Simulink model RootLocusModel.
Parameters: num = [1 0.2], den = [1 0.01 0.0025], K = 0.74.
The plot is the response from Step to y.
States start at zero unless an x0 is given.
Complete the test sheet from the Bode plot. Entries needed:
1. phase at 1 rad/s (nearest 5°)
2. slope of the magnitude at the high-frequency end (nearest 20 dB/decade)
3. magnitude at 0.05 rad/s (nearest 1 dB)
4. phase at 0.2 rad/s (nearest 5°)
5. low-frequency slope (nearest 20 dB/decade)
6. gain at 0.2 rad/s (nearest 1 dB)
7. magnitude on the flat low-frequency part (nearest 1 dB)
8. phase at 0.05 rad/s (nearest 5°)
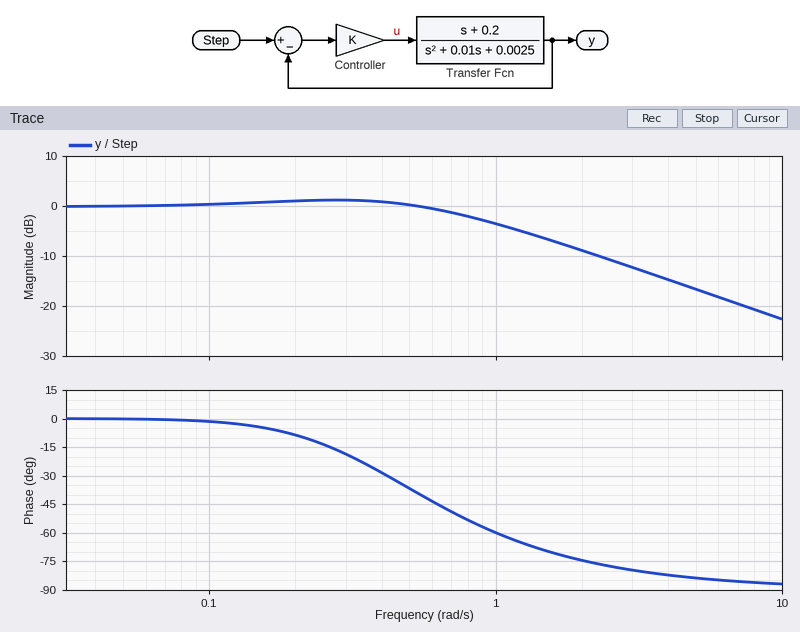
-60°
-20 dB/decade
0 dB
-10°
0 dB/decade
1 dB
0 dB
0°
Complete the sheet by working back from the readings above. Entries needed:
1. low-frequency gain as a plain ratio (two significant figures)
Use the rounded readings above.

1.0
